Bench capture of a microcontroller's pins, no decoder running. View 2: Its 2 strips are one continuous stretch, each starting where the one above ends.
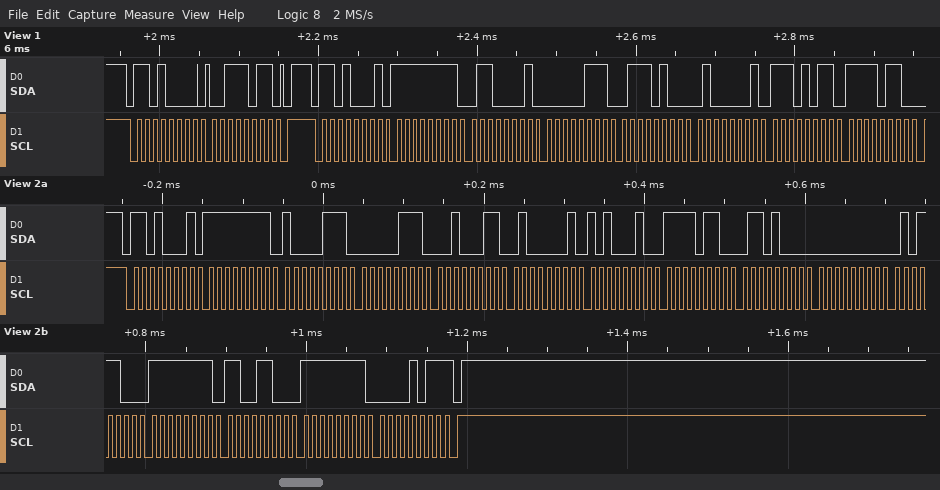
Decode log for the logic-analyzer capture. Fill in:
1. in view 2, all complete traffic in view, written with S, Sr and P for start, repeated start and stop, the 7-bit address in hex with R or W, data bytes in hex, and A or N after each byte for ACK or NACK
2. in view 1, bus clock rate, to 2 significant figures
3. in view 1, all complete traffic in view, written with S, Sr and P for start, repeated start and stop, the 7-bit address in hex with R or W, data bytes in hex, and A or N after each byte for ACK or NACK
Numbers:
S 68R A FF A 87 A 07 A 23 A 41 A A2 A F6 A 68 A 00 A 5C A FF A CC A FF A 0B N P
100 kHz
S 68W A 3B A P S 68R A FF A 61 A 07 A 74 A 41 A EB A F6 A
